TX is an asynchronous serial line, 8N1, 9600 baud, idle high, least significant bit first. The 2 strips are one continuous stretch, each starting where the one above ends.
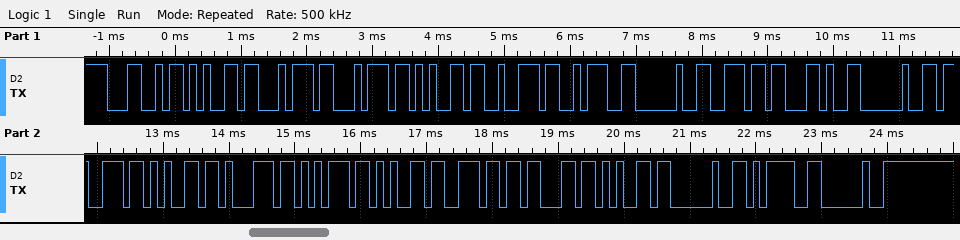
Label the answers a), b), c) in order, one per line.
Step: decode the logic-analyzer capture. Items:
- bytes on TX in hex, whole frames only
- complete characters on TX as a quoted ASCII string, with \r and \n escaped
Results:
a) 4C 65 74 74 65 72 3A 20 6E 2C 20 73 65 71 75 65 6E 63 65 20 3D 20
b) "Letter: n, sequence = "
